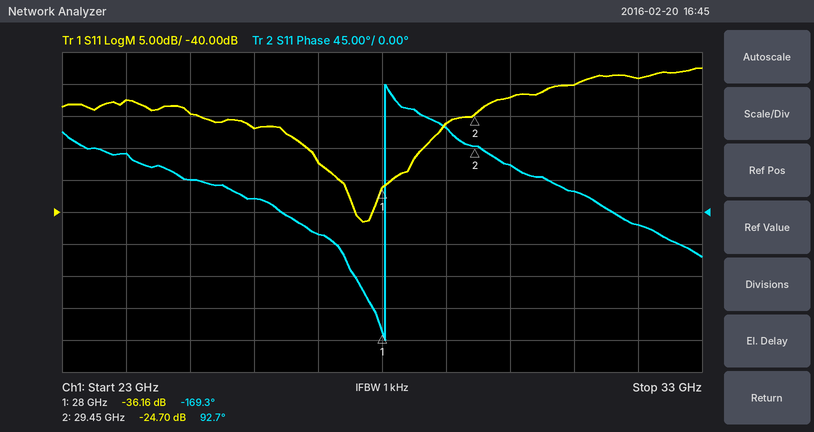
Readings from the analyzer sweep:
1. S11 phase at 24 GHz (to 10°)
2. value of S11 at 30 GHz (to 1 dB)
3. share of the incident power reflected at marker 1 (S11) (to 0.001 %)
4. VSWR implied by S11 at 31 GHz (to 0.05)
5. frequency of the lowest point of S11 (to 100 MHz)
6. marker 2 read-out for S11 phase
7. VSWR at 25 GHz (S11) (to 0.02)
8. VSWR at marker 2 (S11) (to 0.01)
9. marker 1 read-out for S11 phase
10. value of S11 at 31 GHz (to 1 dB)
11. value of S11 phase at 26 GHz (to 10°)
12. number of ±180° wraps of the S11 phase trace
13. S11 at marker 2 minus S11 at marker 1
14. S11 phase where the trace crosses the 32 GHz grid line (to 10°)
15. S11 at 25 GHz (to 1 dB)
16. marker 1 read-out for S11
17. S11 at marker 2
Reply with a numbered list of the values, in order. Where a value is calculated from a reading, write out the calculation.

1. 80°
2. -22 dB
3. 10^(-36.16/10) ≈ 0.024 %
4. |Γ| = 10^(-20/20) = 0.1000; VSWR = (1 + 0.1000)/(1 − 0.1000) ≈ 1.22, so 1.20 to the nearest 0.05
5. 27.7 GHz
6. 92.7°
7. |Γ| = 10^(-25/20) = 0.0562; VSWR = (1 + 0.0562)/(1 − 0.0562) ≈ 1.12
8. (1 + 0.0582)/(1 − 0.0582) ≈ 1.12
9. -169.3°
10. -20 dB
11. 20°
12. 1
13. -24.7 − (-36.16) = 11.46 dB
14. -20°
15. -25 dB
16. -36.16 dB
17. -24.70 dB
